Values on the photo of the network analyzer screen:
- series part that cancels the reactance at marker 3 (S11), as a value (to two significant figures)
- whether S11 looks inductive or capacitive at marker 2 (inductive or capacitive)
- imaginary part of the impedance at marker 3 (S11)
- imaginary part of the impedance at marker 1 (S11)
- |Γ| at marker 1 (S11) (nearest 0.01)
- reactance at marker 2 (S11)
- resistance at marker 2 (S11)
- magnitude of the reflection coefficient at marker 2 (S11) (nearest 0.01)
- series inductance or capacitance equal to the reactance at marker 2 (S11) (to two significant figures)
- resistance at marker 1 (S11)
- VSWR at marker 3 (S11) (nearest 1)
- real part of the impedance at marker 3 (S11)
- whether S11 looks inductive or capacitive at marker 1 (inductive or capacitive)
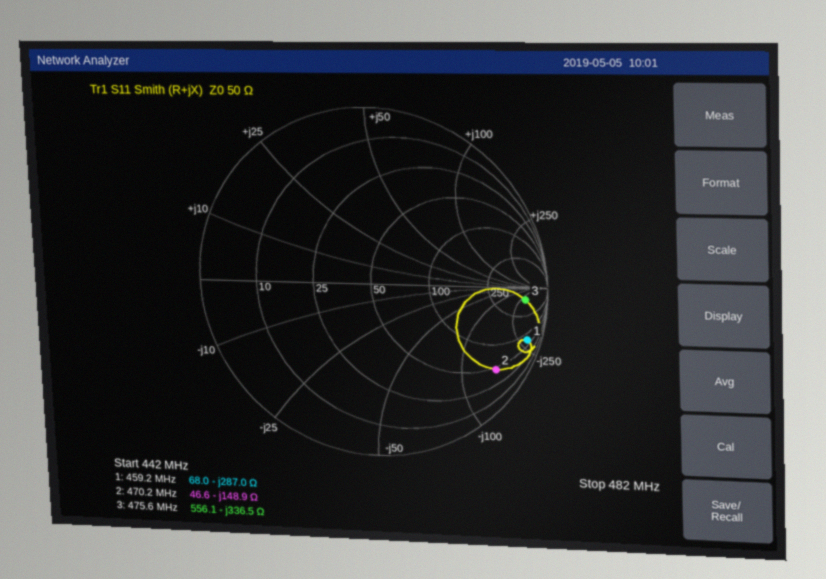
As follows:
110 nH
capacitive
-336.5 Ω
-287.0 Ω
0.93
-148.9 Ω
46.6 Ω
0.84
2.3 pF
68.0 Ω
15
556.1 Ω
capacitive
